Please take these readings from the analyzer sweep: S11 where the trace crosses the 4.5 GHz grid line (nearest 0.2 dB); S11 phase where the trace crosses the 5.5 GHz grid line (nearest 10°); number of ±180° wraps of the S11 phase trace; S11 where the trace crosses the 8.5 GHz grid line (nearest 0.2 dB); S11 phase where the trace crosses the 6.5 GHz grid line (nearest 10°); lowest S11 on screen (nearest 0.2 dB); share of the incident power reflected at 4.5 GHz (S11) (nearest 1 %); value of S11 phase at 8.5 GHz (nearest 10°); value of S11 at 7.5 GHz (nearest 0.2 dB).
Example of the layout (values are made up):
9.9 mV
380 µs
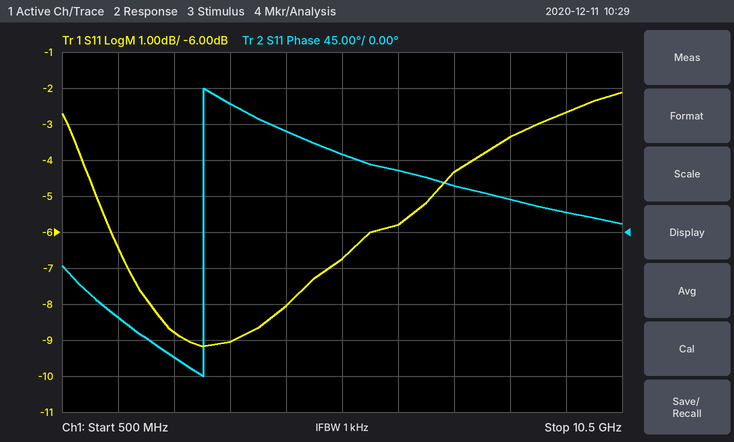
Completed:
-8.0 dB
100°
1
-3.4 dB
80°
-9.2 dB
16 %
40°
-4.4 dB
